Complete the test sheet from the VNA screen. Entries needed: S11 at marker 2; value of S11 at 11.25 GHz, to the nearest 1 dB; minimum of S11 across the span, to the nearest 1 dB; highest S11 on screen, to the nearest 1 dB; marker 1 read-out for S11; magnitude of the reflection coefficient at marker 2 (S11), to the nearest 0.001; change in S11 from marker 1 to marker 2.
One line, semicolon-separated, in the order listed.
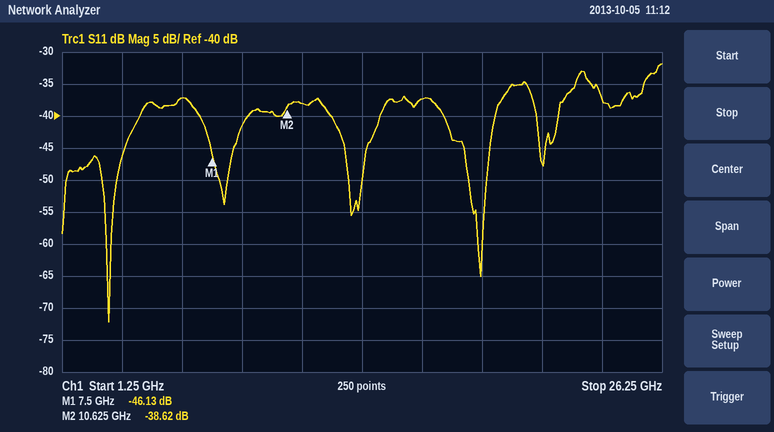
-38.62 dB; -38 dB; -72 dB; -32 dB; -46.13 dB; 0.012; 7.51 dB
